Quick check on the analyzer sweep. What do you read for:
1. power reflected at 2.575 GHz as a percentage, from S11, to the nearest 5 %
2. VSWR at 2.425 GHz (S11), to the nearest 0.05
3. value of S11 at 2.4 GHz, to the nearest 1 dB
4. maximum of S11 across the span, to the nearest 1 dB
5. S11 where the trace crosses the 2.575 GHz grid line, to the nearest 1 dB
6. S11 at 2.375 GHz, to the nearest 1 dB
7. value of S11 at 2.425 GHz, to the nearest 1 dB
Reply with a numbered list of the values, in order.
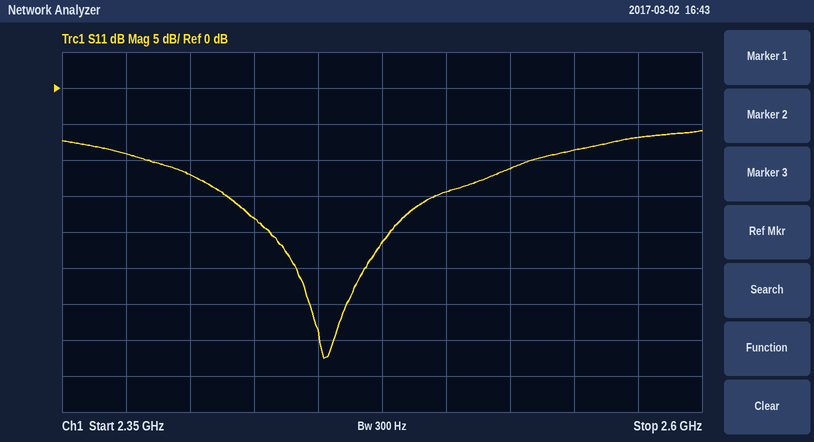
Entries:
1. 20 %
2. 1.30
3. -12 dB
4. -6 dB
5. -7 dB
6. -9 dB
7. -18 dB
